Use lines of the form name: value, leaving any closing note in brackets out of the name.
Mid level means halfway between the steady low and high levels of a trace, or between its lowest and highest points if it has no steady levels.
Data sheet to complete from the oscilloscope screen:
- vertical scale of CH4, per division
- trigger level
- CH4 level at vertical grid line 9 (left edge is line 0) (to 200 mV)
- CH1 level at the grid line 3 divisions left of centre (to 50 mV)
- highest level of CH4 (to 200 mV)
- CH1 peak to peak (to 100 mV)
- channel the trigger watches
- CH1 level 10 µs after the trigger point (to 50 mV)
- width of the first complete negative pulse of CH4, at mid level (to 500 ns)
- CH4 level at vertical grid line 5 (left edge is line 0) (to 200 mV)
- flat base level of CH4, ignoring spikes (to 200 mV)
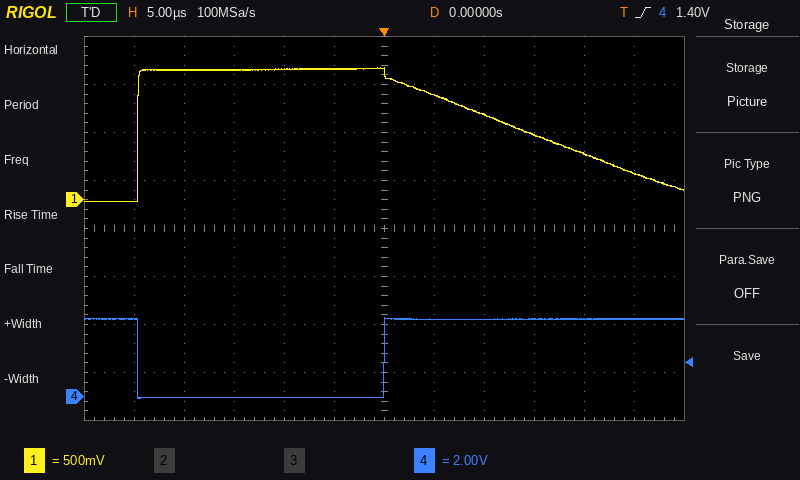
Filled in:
vertical scale of CH4, per division: 2 V
trigger level: 1.40 V
CH4 level at vertical grid line 9 (left edge is line 0): 3.2 V
CH1 level at the grid line 3 divisions left of centre: 1.35 V
highest level of CH4: 3.2 V
CH1 peak to peak: 1.40 V
channel the trigger watches: CH4
CH1 level 10 µs after the trigger point: 900 mV
width of the first complete negative pulse of CH4, at mid level: 24.5 µs
CH4 level at vertical grid line 5 (left edge is line 0): 0.0 V
flat base level of CH4, ignoring spikes: 0.0 V
